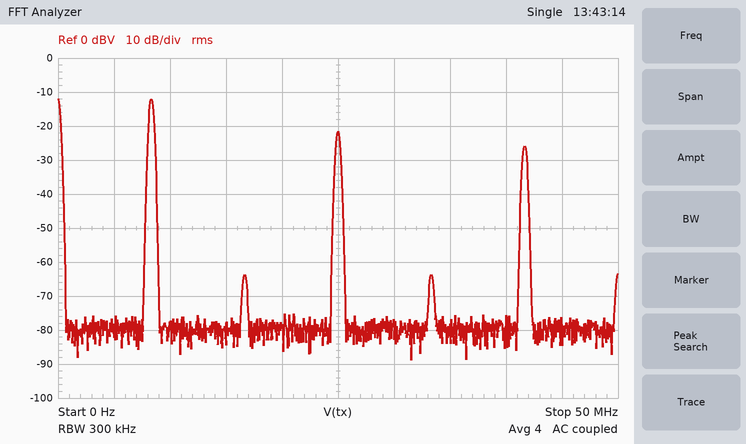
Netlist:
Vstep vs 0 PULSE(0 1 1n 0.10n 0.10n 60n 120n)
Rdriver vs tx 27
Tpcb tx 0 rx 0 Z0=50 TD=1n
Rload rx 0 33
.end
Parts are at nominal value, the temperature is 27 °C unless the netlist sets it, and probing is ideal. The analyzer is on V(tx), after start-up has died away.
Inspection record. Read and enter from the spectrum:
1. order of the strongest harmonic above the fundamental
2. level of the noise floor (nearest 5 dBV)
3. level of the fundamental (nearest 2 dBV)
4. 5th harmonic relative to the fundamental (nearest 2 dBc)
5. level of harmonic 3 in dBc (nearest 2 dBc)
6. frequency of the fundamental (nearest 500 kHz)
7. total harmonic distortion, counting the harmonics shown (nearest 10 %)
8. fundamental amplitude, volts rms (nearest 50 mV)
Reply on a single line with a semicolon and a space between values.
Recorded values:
3; -80 dBV; -12 dBV; -14 dBc; -10 dBc; 8.5 MHz; 40 %; 250 mV
